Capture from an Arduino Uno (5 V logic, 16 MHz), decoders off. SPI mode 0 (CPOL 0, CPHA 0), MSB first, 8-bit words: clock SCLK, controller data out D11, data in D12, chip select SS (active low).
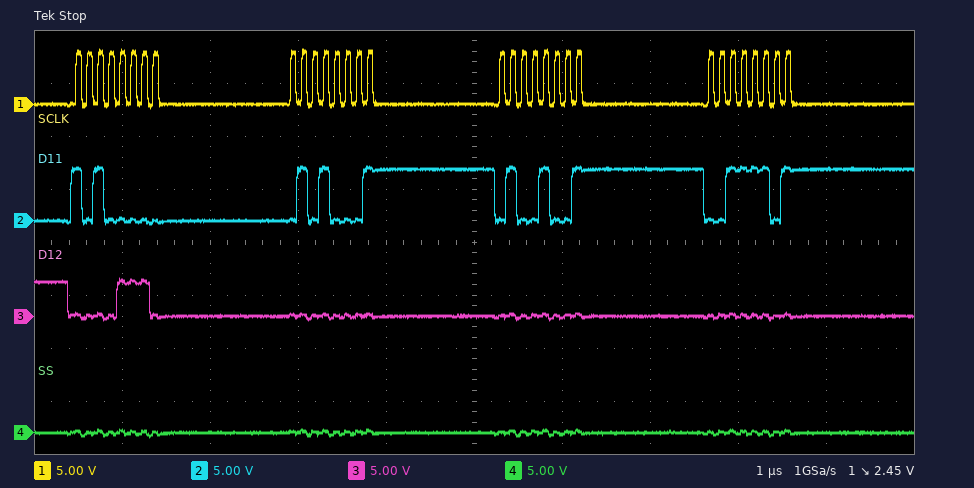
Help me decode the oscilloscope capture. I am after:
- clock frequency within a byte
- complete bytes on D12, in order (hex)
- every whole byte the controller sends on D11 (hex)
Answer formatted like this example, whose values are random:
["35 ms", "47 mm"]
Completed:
["8 MHz", "0E 00 00 00", "A0 51 49 3D"]
